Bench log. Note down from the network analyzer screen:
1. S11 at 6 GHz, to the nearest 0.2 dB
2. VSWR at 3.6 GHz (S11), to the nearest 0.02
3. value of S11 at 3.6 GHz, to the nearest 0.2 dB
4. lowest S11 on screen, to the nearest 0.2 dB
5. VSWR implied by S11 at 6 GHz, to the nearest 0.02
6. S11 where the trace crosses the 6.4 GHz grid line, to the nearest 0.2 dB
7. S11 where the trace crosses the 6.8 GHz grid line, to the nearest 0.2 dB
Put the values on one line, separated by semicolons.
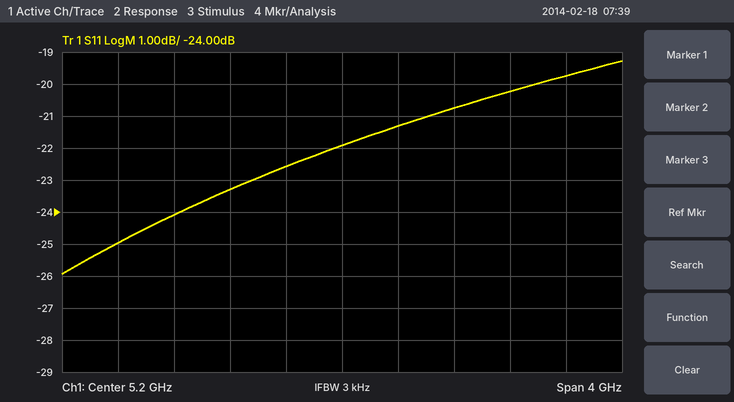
-20.8 dB; 1.12; -25.0 dB; -26.0 dB; 1.20; -20.2 dB; -19.8 dB
